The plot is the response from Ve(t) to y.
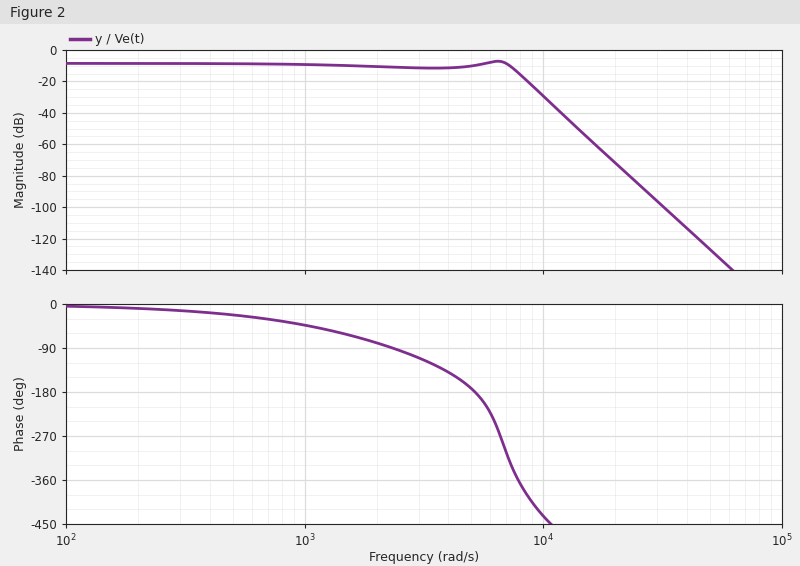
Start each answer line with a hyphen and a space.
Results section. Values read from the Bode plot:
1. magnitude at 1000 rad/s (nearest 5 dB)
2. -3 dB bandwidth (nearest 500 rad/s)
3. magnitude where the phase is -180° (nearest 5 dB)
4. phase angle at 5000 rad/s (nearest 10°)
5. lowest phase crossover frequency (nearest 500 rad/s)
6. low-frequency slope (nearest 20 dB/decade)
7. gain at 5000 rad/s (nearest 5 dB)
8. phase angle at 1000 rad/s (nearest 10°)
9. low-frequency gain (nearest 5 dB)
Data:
- -10 dB
- 7500 rad/s
- -10 dB
- -170°
- 5000 rad/s
- 0 dB/decade
- -10 dB
- -40°
- -10 dB
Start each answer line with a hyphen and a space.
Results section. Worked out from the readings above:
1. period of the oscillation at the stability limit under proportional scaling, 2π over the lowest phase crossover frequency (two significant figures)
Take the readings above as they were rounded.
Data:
- 0.0013 s
